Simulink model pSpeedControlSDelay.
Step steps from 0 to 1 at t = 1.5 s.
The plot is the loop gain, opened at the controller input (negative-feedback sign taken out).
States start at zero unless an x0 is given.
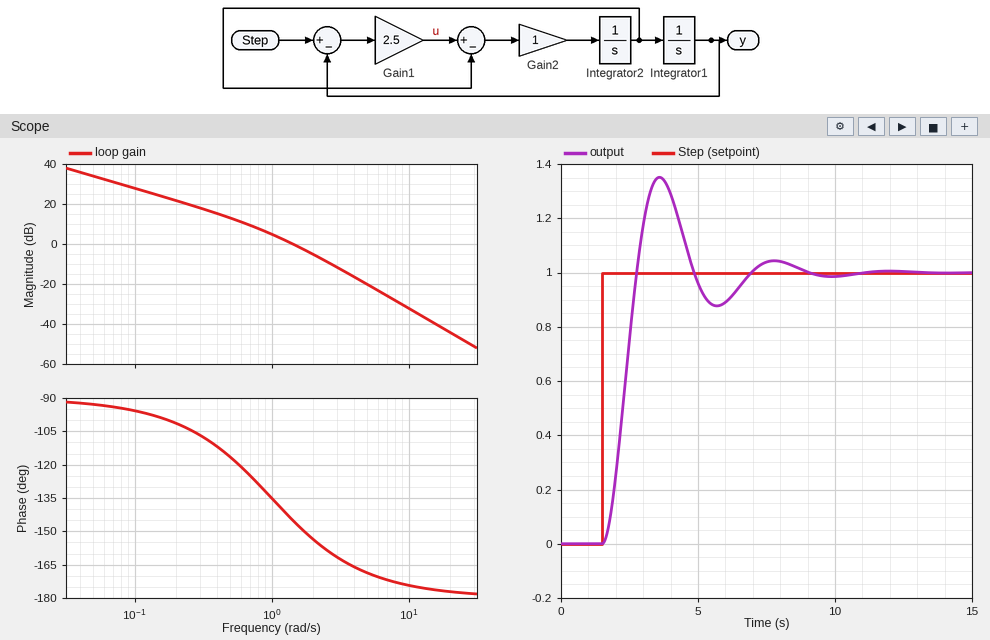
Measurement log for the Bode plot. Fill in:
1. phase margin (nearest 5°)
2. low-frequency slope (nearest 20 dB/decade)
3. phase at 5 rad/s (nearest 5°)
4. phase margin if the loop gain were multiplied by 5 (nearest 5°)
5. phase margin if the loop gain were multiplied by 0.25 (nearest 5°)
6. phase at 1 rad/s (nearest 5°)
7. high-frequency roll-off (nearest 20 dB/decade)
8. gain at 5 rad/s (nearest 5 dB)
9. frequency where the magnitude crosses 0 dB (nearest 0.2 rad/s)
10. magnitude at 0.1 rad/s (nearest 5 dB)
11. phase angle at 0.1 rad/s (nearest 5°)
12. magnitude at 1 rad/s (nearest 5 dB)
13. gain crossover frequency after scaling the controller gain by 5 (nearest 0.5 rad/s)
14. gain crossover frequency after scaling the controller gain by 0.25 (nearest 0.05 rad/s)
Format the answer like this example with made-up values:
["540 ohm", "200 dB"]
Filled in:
["35°", "-20 dB/decade", "-170°", "15°", "60°", "-135°", "-40 dB/decade", "-20 dB", "1.4 rad/s", "30 dB", "-95°", "5 dB", "3.5 rad/s", "0.55 rad/s"]
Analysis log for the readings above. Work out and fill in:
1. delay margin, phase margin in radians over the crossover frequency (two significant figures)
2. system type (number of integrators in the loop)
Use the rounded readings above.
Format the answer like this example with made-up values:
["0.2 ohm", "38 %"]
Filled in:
["0.44 s", "1"]
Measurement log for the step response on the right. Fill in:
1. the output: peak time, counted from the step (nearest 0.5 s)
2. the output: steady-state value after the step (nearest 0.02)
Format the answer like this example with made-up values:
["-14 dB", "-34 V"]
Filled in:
["2.0 s", "1.00"]
